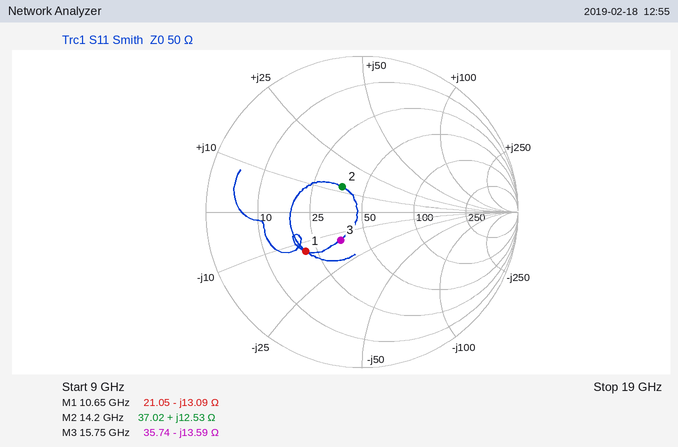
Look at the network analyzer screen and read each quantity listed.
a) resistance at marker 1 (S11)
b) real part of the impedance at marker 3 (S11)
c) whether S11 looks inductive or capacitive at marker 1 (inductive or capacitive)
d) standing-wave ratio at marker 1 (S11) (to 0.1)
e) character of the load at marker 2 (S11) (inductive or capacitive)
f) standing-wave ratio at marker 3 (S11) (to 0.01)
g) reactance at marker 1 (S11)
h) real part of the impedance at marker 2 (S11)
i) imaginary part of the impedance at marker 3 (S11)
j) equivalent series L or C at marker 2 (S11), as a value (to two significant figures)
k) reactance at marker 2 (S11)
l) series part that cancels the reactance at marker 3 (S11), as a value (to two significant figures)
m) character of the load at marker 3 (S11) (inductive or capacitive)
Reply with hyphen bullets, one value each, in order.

- 21.05 Ω
- 35.74 Ω
- capacitive
- 2.6
- inductive
- 1.59
- -13.09 Ω
- 37.02 Ω
- -13.59 Ω
- 140 pH
- +12.53 Ω
- 140 pH
- capacitive
